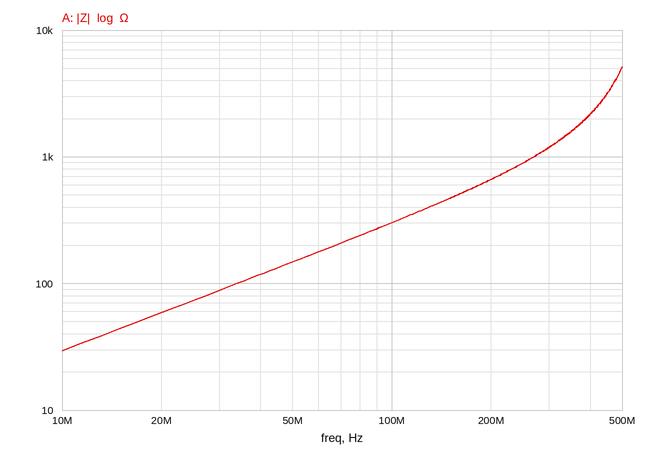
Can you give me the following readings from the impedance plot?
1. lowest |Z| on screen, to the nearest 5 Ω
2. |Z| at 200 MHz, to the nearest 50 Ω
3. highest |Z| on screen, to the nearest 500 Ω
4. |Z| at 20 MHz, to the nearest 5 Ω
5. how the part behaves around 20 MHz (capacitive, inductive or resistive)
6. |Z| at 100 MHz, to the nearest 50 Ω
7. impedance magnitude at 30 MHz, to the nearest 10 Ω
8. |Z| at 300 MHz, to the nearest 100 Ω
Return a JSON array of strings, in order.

["30 Ω", "650 Ω", "5.0 kΩ", "60 Ω", "inductive", "300 Ω", "90 Ω", "1.2 kΩ"]
